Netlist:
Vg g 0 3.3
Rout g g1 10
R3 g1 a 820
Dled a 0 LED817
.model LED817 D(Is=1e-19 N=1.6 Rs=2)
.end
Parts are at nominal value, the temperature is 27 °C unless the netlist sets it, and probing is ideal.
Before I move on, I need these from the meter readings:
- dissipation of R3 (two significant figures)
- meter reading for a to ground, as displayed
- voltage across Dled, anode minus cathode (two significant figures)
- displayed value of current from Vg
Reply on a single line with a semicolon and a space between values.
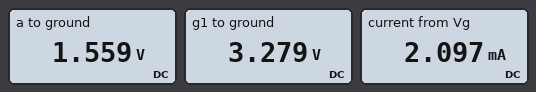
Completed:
3.6 mW; 1.559 V; 1.6 V; 2.097 mA
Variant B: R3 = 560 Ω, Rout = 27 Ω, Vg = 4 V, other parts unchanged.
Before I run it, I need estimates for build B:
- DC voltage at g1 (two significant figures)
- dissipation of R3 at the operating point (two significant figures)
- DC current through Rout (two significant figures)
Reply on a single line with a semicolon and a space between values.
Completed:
3.9 V; 9.4 mW; 4.1 mA
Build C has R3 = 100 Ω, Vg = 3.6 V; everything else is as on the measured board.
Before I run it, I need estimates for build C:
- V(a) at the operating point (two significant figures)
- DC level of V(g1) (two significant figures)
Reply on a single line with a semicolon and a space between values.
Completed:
1.7 V; 3.4 V
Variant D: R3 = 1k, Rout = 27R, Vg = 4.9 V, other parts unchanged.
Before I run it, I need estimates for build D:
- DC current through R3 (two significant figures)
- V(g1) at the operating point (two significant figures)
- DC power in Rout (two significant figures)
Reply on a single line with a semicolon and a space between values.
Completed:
3.2 mA; 4.8 V; 280 µW
